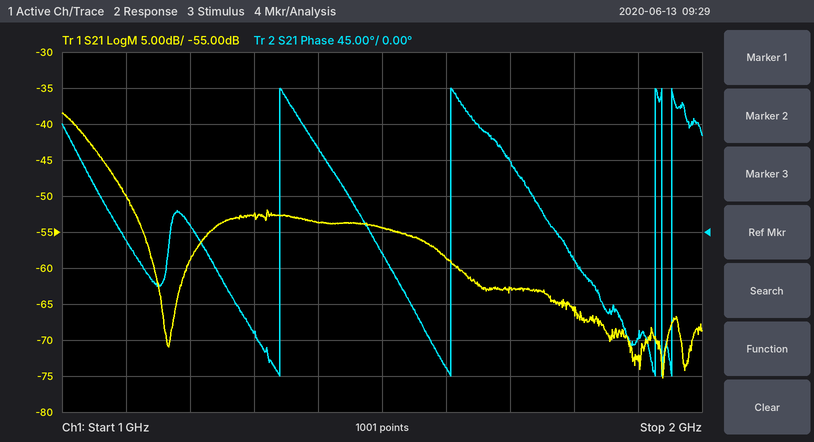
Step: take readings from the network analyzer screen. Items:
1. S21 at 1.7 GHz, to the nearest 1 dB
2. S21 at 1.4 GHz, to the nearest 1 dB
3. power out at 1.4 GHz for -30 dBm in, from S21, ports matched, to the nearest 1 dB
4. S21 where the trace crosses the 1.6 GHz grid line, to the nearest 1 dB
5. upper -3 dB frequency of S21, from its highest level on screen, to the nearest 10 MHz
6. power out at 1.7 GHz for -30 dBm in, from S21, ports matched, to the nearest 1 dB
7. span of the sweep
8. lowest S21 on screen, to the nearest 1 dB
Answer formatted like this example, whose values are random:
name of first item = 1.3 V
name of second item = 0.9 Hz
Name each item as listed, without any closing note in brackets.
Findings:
S21 at 1.7 GHz, to the nearest 1 dB = -63 dB
S21 at 1.4 GHz, to the nearest 1 dB = -54 dB
power out at 1.4 GHz for -30 dBm in, from S21, ports matched, to the nearest 1 dB = -84 dBm
S21 where the trace crosses the 1.6 GHz grid line, to the nearest 1 dB = -59 dB
upper -3 dB frequency of S21, from its highest level on screen, to the nearest 10 MHz = 1.03 GHz
power out at 1.7 GHz for -30 dBm in, from S21, ports matched, to the nearest 1 dB = -93 dBm
span of the sweep = 1 GHz
lowest S21 on screen, to the nearest 1 dB = -75 dB
